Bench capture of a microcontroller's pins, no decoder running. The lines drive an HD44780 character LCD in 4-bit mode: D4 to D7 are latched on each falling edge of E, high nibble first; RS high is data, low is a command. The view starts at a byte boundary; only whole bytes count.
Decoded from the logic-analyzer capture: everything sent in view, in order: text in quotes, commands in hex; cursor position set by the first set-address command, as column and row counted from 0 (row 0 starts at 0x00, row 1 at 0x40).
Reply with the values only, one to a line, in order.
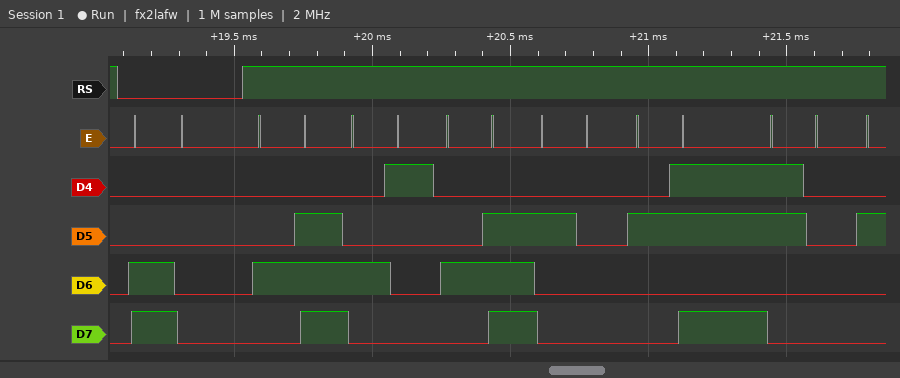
0xC0 "NAN +0"
column 0, row 1
